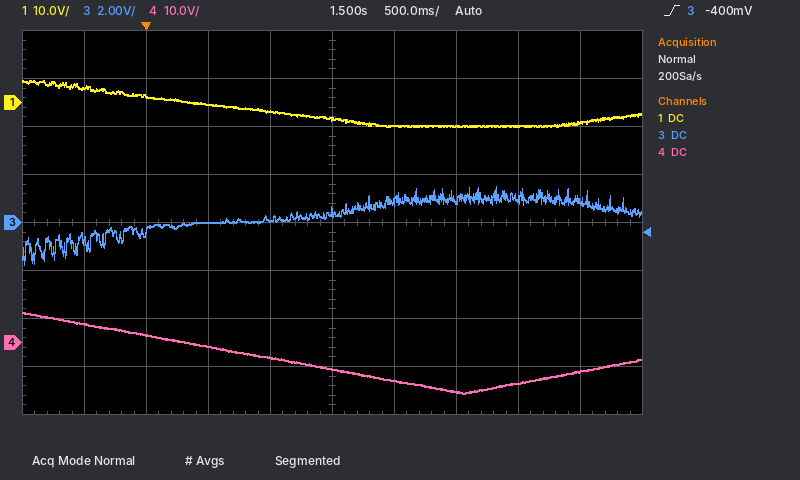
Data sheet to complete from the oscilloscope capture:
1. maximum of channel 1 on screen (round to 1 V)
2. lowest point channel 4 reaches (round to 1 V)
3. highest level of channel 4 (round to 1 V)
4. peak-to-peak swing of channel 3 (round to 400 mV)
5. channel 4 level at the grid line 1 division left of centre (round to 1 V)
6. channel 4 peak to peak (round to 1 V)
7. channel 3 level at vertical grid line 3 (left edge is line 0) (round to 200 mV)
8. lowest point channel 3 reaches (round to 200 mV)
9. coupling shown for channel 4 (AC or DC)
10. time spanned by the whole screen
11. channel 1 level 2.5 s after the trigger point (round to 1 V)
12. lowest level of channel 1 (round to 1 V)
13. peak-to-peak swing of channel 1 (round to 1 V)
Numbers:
5 V
-11 V
6 V
3.2 V
-3 V
17 V
0.0 V
-1.8 V
DC
5 s
-5 V
-5 V
10 V
